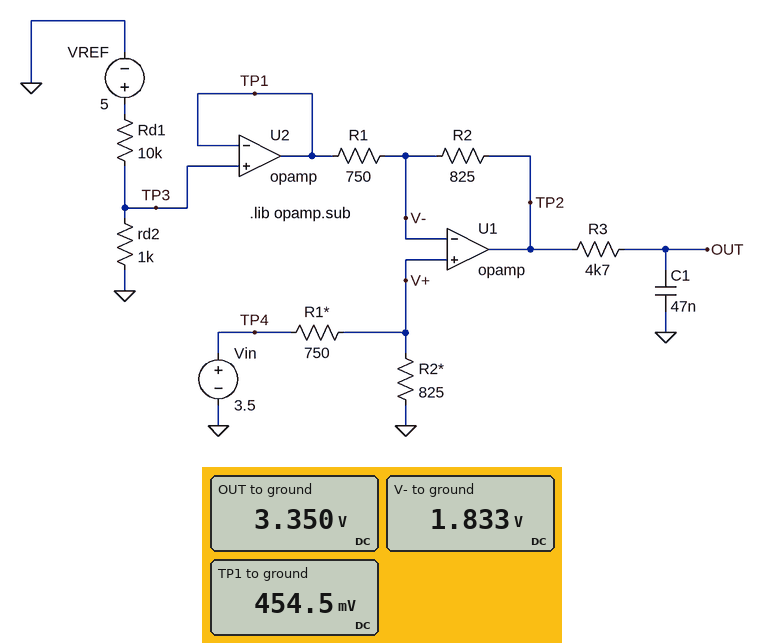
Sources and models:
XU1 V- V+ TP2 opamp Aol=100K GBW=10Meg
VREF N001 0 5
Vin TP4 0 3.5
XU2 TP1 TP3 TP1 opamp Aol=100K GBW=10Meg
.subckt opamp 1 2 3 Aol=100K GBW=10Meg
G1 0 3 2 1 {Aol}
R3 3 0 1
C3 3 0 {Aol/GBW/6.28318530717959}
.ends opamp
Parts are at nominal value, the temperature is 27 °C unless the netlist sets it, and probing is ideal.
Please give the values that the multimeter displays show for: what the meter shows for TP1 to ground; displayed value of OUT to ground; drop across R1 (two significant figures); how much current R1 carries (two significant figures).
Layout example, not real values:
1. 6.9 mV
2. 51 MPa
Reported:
1. 454.5 mV
2. 3.350 V
3. 1.4 V
4. 1.8 mA
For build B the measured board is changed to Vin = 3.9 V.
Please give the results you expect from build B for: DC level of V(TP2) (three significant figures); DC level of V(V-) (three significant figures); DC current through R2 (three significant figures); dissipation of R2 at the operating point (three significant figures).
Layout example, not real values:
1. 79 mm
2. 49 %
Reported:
1. 3.79 V
2. 2.04 V
3. 2.12 mA
4. 3.70 mW
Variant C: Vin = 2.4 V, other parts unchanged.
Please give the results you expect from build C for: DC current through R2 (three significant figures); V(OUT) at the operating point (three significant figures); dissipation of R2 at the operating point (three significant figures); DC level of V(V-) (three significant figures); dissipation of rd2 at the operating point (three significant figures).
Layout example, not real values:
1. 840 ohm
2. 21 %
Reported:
1. 1.07 mA
2. 2.14 V
3. 945 µW
4. 1.26 V
5. 207 µW
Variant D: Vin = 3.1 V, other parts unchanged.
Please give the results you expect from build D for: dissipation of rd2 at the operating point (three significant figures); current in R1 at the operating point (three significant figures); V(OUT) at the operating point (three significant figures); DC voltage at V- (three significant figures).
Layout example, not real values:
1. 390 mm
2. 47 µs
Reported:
1. 207 µW
2. 1.56 mA
3. 2.91 V
4. 1.62 V
